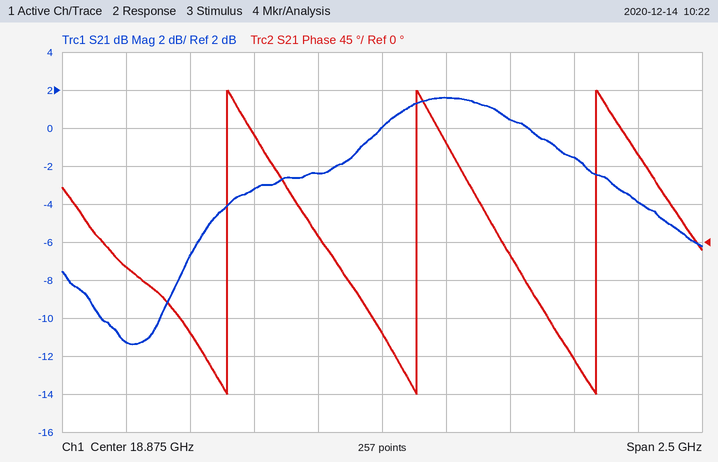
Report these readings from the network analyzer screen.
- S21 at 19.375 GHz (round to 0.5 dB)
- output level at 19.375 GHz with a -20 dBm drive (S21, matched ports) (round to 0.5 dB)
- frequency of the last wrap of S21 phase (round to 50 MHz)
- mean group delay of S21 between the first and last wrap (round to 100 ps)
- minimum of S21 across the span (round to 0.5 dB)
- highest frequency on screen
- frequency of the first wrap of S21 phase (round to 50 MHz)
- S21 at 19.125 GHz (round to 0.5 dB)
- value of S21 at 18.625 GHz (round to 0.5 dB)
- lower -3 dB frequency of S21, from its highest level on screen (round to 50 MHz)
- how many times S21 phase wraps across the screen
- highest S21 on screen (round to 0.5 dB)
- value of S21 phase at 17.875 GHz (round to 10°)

0.5 dB
-19.5 dBm
19.70 GHz
1.4 ns
-11.5 dB
20.125 GHz
18.25 GHz
1.5 dB
-2.5 dB
18.75 GHz
3
1.5 dB
-30°
